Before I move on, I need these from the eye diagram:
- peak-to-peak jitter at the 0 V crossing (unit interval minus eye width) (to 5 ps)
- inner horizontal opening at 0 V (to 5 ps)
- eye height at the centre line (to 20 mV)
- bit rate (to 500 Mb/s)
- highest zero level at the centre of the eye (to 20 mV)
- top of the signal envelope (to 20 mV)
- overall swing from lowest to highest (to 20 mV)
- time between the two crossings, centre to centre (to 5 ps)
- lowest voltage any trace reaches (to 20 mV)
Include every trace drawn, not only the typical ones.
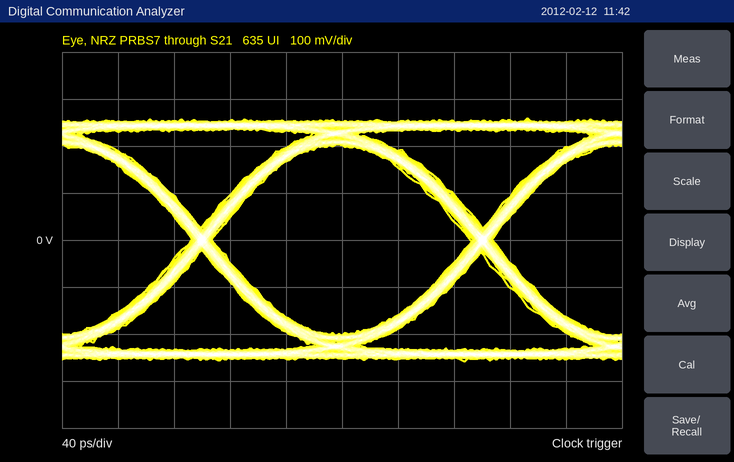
15 ps
185 ps
400 mV
5.0 Gb/s
-200 mV
260 mV
520 mV
200 ps
-260 mV
